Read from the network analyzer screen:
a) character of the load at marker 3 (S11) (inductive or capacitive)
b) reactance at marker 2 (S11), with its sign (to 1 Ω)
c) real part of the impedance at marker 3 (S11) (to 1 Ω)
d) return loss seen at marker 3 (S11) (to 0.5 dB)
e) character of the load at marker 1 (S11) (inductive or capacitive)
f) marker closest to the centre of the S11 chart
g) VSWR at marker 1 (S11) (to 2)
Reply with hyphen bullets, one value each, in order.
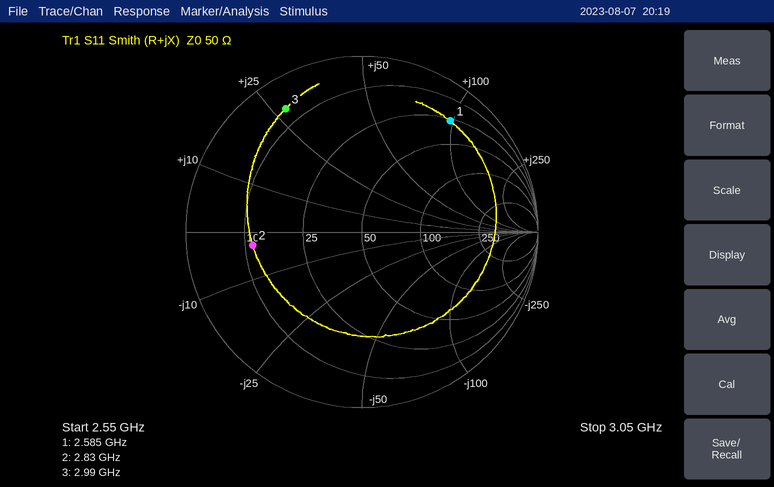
- inductive
- -3 Ω
- 6 Ω
- 1.5 dB
- inductive
- marker 2
- 10
